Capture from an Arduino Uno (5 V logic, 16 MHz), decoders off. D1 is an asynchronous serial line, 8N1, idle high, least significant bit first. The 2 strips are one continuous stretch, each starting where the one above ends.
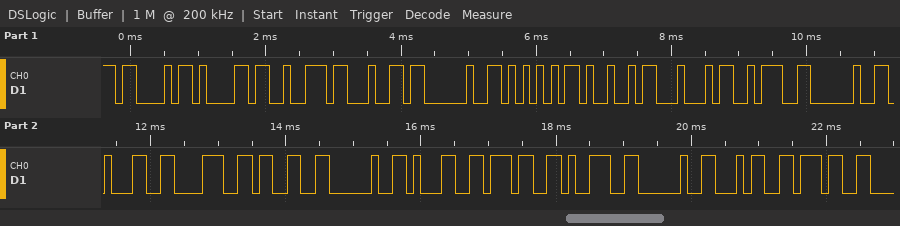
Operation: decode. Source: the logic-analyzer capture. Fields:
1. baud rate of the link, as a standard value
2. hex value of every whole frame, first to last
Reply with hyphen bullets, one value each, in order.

- 9600 baud
- 43 61 72 64 20 55 49 44 3A 20 31 38 33 20 31 37 39 20 34 37
